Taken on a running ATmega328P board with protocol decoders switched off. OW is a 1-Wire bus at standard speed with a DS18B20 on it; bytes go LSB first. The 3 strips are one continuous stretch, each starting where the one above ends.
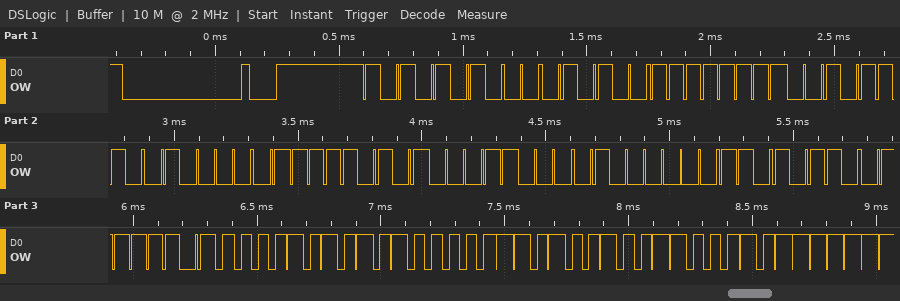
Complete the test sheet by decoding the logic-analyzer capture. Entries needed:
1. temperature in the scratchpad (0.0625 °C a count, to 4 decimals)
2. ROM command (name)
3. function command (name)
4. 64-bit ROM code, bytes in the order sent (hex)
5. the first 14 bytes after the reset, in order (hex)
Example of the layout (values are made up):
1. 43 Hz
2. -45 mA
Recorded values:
1. 85.0000 °C
2. Match ROM
3. Read Scratchpad
4. 28 FF 74 82 AF 18 02 6B
5. 55 28 FF 74 82 AF 18 02 6B BE 50 05 4B 46
